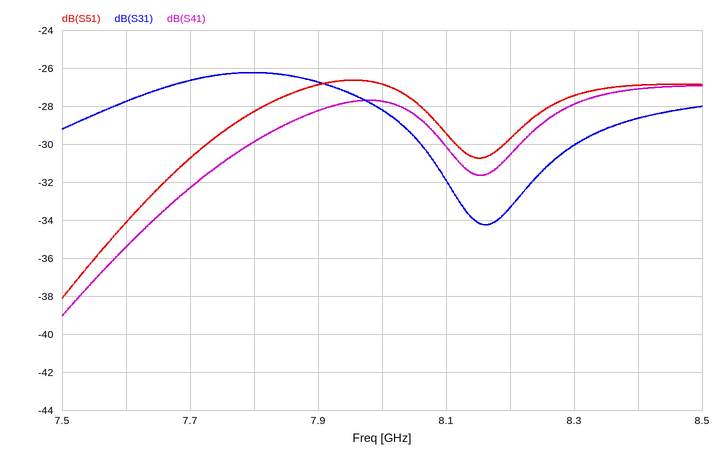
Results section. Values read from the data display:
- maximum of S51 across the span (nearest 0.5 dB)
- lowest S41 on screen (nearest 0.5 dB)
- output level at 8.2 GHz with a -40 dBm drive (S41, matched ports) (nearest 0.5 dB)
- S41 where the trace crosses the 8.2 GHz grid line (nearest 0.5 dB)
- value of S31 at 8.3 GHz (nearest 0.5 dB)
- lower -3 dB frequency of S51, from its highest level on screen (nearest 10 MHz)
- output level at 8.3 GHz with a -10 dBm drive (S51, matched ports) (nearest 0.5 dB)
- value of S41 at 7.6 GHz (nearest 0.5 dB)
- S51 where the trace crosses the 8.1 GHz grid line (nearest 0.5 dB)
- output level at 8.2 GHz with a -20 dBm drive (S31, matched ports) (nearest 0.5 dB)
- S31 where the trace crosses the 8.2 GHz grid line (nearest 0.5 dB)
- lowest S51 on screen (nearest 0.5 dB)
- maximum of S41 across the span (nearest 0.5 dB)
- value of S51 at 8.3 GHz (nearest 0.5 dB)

-26.5 dB
-39.0 dB
-70.5 dBm
-30.5 dB
-30.0 dB
7.74 GHz
-37.5 dBm
-35.5 dB
-29.5 dB
-53.5 dBm
-33.5 dB
-38.0 dB
-27.0 dB
-27.5 dB
